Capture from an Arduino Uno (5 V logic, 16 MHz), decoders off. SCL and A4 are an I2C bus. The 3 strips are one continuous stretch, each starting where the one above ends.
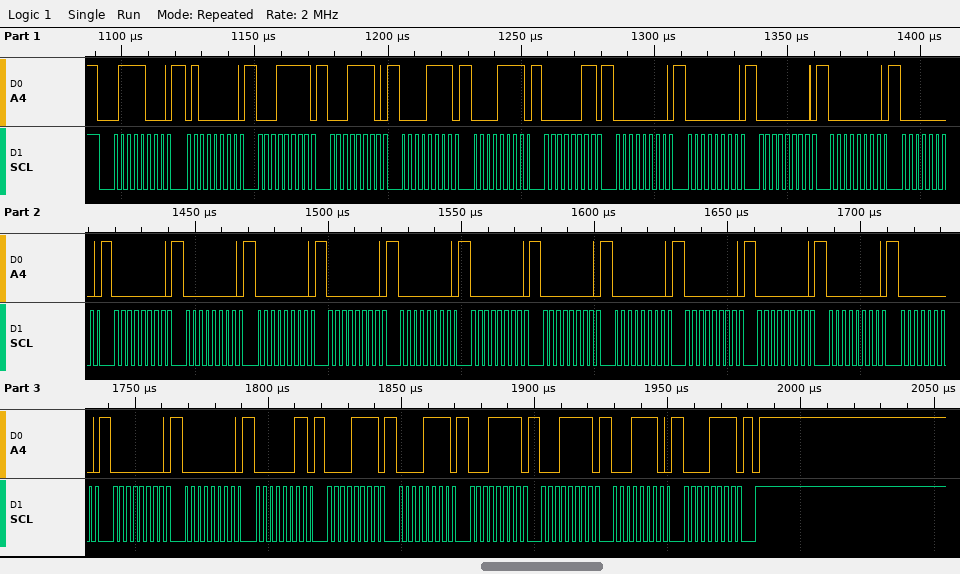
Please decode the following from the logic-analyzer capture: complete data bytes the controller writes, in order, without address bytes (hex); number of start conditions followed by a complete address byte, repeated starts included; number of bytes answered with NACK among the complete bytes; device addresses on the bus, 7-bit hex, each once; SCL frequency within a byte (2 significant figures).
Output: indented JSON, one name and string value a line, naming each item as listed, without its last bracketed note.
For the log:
{
  "complete data bytes the controller writes, in order, without address bytes": "40 1F 1E 0F 0F 03 00 00 00 00 00 00 00 00 00 00 00 00 00 00 00 00 00 00 00 03 0F 0F 1F 1F 1E 0F",
  "number of start conditions followed by a complete address byte, repeated starts included": "1",
  "number of bytes answered with NACK among the complete bytes": "0",
  "device addresses on the bus, 7-bit hex, each once": "0x3C",
  "SCL frequency within a byte": "400 kHz"
}
